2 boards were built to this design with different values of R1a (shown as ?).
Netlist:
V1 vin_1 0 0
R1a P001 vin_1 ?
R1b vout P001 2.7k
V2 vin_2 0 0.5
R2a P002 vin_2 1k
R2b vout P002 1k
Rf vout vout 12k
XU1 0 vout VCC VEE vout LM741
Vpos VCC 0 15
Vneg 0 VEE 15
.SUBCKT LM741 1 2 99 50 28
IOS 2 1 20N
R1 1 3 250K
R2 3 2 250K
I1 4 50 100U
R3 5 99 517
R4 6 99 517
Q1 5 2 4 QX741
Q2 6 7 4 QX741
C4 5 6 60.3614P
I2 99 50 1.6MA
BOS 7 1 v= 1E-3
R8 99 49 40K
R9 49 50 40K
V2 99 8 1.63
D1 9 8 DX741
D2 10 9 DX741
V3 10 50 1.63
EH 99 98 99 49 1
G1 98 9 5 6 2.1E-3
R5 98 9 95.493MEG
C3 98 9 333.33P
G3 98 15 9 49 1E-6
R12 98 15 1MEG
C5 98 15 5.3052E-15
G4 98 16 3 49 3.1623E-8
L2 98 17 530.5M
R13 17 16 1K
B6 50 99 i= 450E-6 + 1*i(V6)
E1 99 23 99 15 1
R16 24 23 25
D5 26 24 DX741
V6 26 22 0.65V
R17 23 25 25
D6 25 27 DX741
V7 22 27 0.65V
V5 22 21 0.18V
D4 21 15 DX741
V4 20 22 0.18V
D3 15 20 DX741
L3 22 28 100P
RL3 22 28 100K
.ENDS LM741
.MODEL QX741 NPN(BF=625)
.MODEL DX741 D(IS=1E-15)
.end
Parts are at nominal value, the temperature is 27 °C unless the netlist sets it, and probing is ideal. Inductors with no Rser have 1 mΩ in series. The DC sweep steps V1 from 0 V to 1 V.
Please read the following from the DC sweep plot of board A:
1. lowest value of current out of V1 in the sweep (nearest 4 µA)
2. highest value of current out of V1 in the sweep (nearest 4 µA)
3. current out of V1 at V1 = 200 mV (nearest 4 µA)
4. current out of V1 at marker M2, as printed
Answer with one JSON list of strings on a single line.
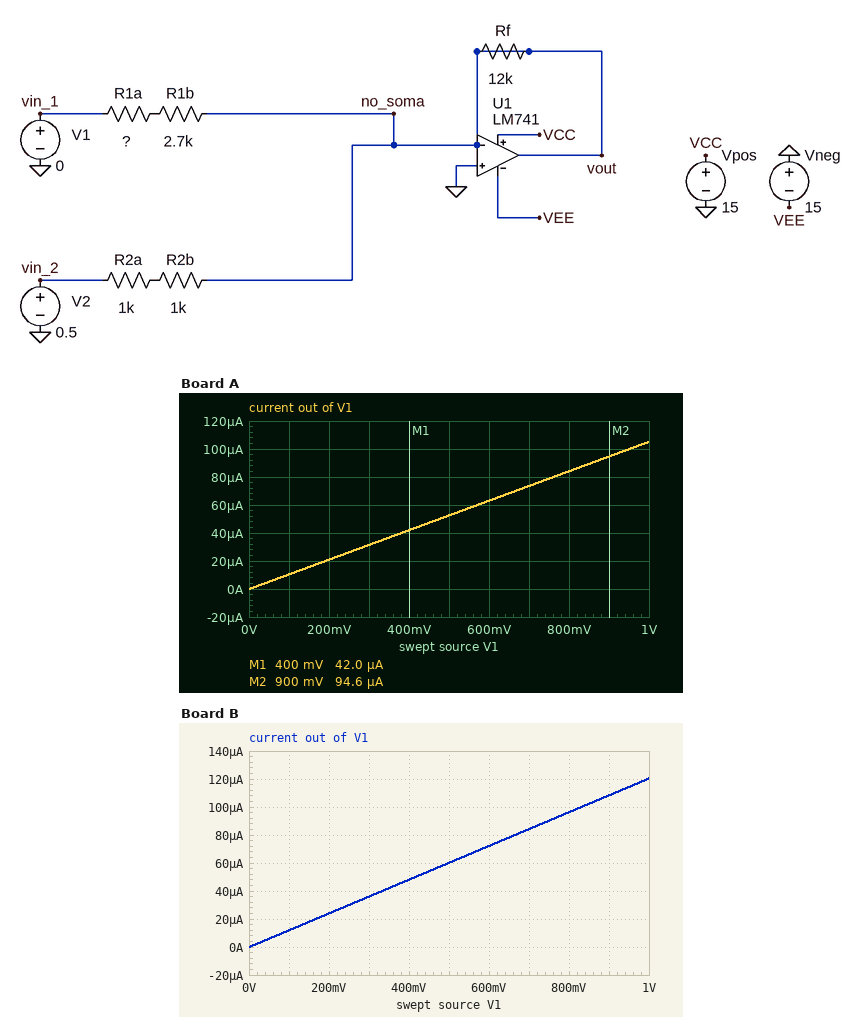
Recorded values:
["0 A", "104 µA", "20 µA", "94.6 µA"]
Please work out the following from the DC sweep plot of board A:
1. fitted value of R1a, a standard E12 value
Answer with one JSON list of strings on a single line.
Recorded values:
["6.8 kΩ"]
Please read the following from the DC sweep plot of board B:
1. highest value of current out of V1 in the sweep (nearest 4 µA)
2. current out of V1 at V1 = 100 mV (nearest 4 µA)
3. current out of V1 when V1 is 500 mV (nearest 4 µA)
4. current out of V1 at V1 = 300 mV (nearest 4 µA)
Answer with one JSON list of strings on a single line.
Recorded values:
["120 µA", "12 µA", "60 µA", "36 µA"]
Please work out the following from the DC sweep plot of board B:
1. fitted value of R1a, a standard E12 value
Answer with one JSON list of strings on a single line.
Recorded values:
["5.6 kΩ"]
